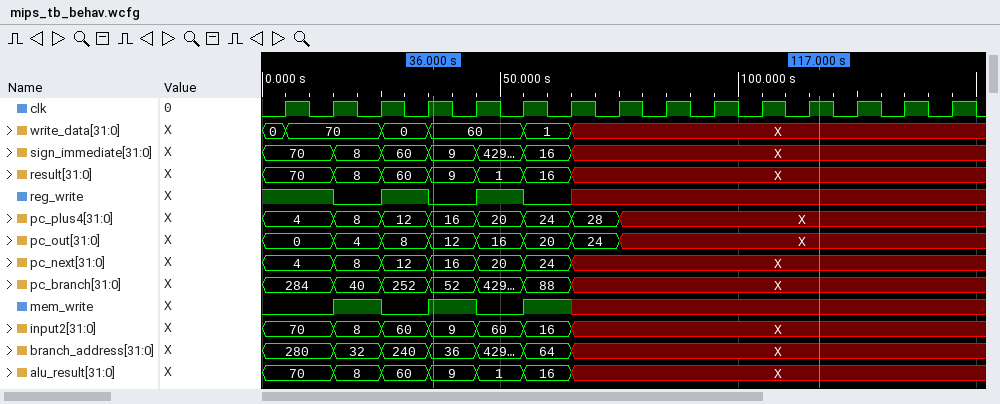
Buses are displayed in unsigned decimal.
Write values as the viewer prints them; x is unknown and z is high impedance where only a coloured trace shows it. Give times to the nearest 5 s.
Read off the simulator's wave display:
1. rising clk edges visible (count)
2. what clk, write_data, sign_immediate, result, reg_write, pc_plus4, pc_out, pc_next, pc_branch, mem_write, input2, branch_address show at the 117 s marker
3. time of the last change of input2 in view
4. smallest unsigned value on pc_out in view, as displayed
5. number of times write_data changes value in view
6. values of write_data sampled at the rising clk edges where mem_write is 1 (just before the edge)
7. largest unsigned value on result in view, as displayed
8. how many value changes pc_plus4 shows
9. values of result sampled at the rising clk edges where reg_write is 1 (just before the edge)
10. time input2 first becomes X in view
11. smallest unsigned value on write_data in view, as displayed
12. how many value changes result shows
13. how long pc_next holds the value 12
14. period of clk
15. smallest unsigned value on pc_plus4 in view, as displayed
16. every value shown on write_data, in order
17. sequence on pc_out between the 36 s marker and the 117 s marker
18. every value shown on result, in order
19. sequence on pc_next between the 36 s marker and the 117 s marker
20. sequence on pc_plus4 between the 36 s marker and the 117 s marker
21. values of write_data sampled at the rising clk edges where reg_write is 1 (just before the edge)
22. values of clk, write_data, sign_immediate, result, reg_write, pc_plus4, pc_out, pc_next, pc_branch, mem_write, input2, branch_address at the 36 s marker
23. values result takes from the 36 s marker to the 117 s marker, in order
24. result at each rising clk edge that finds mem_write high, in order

15
clk=1, write_data=X, sign_immediate=X, result=X, reg_write=x, pc_plus4=X, pc_out=X, pc_next=X, pc_branch=X, mem_write=x, input2=X, branch_address=X
65 s
0
5
70, 60, 1
70
7
70, 70, 60, 1
65 s
0
6
10 s
10 s
4
0, 70, 0, 60, 1, X
12, 16, 20, 24, X
70, 8, 60, 9, 1, 16, X
16, 20, 24, X
16, 20, 24, 28, X
0, 70, 0, 60
clk=1, write_data=60, sign_immediate=9, result=9, reg_write=0, pc_plus4=16, pc_out=12, pc_next=16, pc_branch=52, mem_write=1, input2=9, branch_address=36
9, 1, 16, X
8, 9, 16
